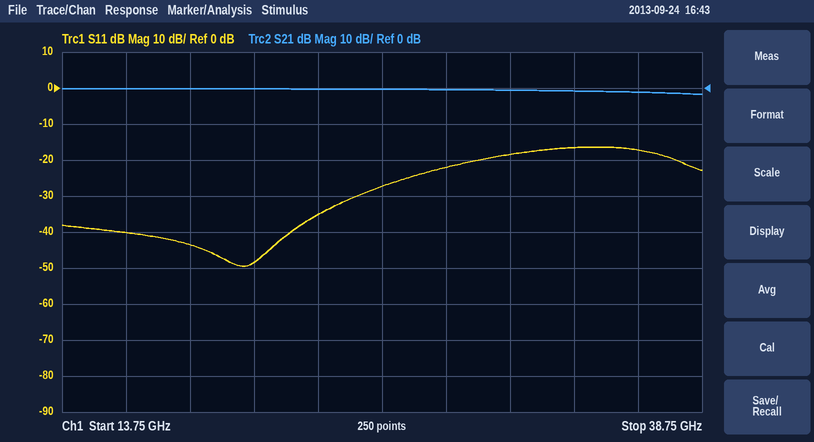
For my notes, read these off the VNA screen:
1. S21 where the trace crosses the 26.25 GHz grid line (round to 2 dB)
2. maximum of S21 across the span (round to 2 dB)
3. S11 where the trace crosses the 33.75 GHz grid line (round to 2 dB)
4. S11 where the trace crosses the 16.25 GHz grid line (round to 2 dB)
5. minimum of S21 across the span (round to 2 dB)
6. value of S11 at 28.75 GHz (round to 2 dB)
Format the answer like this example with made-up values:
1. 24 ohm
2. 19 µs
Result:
1. 0 dB
2. 0 dB
3. -16 dB
4. -40 dB
5. -2 dB
6. -22 dB
